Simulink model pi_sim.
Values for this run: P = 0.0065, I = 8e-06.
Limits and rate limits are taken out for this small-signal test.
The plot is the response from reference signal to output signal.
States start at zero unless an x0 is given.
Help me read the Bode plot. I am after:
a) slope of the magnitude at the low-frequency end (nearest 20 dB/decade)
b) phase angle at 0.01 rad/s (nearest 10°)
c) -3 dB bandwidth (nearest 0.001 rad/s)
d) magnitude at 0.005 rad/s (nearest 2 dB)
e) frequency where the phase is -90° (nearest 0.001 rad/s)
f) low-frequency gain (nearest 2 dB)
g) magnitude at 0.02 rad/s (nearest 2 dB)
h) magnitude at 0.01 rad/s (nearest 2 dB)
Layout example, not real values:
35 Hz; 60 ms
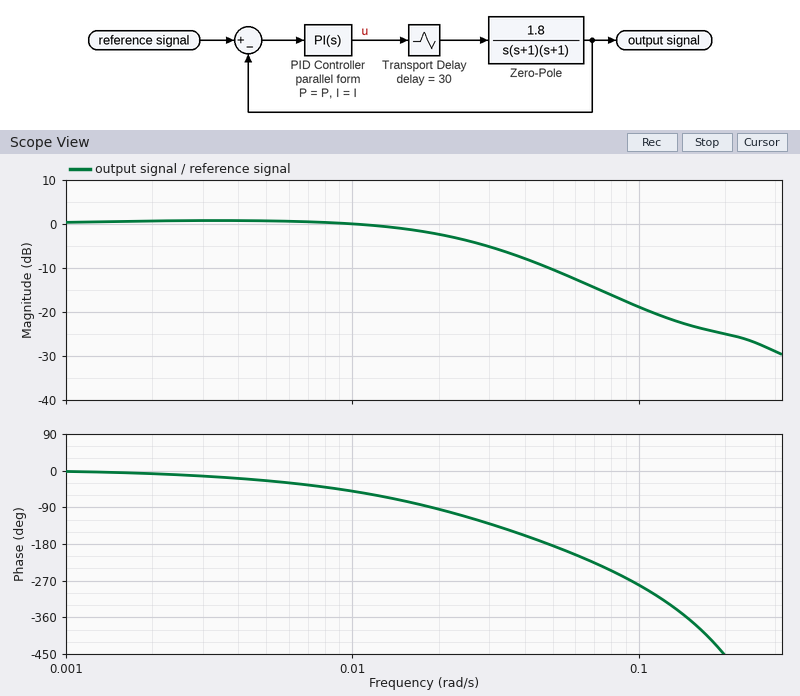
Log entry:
0 dB/decade; -50°; 0.021 rad/s; 0 dB; 0.019 rad/s; 0 dB; -2 dB; 0 dB
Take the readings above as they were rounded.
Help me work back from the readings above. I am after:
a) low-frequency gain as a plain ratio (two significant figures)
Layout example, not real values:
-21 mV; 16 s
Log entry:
1.0
